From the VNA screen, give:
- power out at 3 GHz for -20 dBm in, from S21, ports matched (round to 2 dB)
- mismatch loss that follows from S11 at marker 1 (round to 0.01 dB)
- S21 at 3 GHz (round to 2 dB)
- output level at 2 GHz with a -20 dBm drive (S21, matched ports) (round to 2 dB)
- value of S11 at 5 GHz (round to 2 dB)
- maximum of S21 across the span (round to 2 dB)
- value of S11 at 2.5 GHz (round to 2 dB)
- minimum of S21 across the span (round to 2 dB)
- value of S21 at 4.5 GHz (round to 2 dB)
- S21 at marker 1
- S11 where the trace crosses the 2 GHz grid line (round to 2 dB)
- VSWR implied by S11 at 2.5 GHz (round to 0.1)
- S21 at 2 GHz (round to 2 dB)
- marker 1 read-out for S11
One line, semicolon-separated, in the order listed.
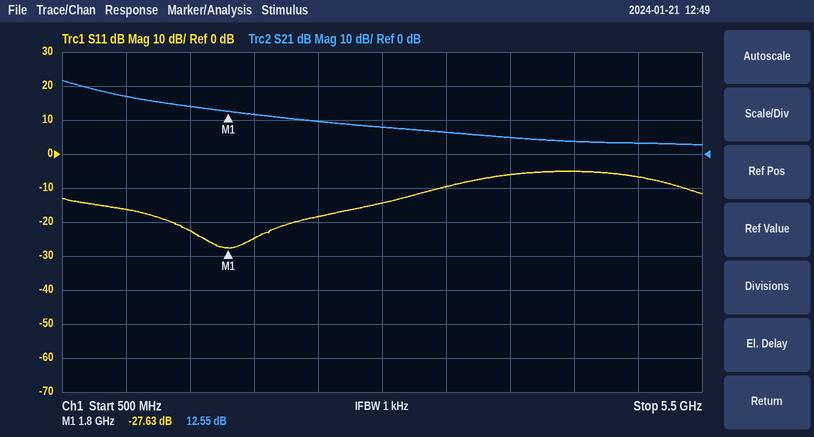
-12 dBm; 0.01 dB; 8 dB; -8 dBm; -6 dB; 22 dB; -18 dB; 2 dB; 4 dB; 12.55 dB; -24 dB; 1.3; 12 dB; -27.63 dB
